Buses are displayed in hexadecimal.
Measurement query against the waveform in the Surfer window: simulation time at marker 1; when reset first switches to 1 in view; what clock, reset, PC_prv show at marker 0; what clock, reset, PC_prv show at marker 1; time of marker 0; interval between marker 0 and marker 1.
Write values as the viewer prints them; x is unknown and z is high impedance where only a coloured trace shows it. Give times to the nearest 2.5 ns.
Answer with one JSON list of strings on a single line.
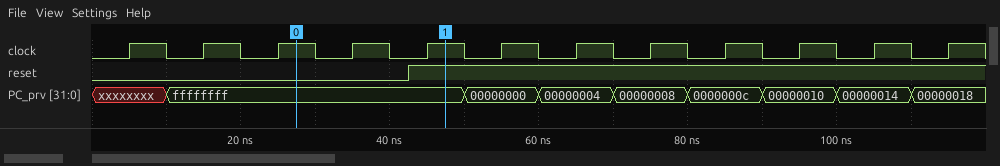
["47.5 ns", "42.5 ns", "clock=1, reset=0, PC_prv=ffffffff", "clock=1, reset=1, PC_prv=ffffffff", "27.5 ns", "20 ns"]
